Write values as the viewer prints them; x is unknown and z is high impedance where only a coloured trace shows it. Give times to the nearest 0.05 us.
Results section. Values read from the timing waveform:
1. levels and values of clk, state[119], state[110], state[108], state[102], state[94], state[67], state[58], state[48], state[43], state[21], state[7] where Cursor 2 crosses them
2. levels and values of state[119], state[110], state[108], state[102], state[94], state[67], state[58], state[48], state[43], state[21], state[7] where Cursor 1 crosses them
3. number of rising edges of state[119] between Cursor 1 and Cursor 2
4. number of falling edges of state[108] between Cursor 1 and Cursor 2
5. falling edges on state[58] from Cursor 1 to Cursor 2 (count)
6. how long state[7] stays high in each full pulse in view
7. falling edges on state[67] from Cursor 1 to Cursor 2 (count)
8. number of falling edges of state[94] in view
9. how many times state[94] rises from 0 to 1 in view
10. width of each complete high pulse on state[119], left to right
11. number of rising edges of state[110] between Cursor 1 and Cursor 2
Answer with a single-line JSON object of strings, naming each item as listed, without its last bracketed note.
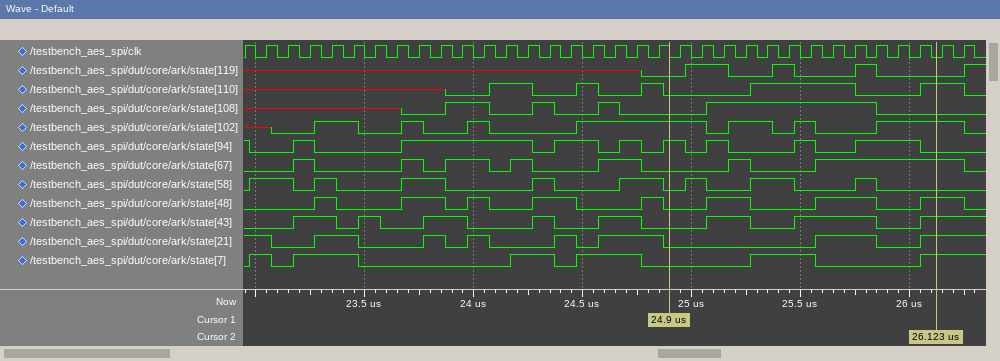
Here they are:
{"levels and values of clk, state[119], state[110], state[108], state[102], state[94], state[67], state[58], state[48], state[43], state[21], state[7] where Cursor 2 crosses them": "clk=0, state[119]=0, state[110]=1, state[108]=0, state[102]=1, state[94]=0, state[67]=1, state[58]=0, state[48]=1, state[43]=1, state[21]=1, state[7]=1", "levels and values of state[119], state[110], state[108], state[102], state[94], state[67], state[58], state[48], state[43], state[21], state[7] where Cursor 1 crosses them": "state[119]=0, state[110]=0, state[108]=0, state[102]=1, state[94]=1, state[67]=0, state[58]=0, state[48]=0, state[43]=0, state[21]=0, state[7]=0", "number of rising edges of state[119] between Cursor 1 and Cursor 2": "3", "number of falling edges of state[108] between Cursor 1 and Cursor 2": "1", "falling edges on state[58] from Cursor 1 to Cursor 2": "3", "how long state[7] stays high in each full pulse in view": "0.1 us, 0.3 us, 0.2 us, 0.3 us, 0.3 us", "falling edges on state[67] from Cursor 1 to Cursor 2": "1", "number of falling edges of state[94] in view": "9", "how many times state[94] rises from 0 to 1 in view": "8", "width of each complete high pulse on state[119], left to right": "0.2 us, 0.1 us, 0.1 us", "number of rising edges of state[110] between Cursor 1 and Cursor 2": "2"}
